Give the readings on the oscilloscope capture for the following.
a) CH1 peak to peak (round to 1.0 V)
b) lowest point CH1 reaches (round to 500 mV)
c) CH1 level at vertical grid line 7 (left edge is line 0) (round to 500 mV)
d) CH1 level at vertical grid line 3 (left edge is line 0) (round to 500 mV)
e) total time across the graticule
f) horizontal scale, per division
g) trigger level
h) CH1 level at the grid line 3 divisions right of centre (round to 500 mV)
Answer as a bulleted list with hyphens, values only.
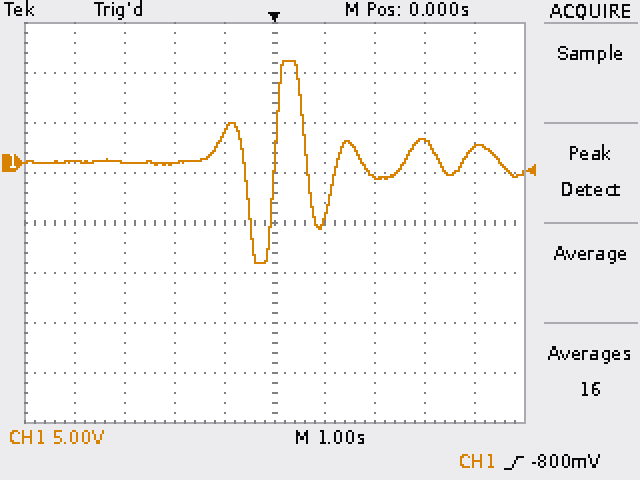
- 20.0 V
- -10.0 V
- -1.5 V
- 0.0 V
- 10 s
- 1 s
- -800 mV
- 2.5 V
